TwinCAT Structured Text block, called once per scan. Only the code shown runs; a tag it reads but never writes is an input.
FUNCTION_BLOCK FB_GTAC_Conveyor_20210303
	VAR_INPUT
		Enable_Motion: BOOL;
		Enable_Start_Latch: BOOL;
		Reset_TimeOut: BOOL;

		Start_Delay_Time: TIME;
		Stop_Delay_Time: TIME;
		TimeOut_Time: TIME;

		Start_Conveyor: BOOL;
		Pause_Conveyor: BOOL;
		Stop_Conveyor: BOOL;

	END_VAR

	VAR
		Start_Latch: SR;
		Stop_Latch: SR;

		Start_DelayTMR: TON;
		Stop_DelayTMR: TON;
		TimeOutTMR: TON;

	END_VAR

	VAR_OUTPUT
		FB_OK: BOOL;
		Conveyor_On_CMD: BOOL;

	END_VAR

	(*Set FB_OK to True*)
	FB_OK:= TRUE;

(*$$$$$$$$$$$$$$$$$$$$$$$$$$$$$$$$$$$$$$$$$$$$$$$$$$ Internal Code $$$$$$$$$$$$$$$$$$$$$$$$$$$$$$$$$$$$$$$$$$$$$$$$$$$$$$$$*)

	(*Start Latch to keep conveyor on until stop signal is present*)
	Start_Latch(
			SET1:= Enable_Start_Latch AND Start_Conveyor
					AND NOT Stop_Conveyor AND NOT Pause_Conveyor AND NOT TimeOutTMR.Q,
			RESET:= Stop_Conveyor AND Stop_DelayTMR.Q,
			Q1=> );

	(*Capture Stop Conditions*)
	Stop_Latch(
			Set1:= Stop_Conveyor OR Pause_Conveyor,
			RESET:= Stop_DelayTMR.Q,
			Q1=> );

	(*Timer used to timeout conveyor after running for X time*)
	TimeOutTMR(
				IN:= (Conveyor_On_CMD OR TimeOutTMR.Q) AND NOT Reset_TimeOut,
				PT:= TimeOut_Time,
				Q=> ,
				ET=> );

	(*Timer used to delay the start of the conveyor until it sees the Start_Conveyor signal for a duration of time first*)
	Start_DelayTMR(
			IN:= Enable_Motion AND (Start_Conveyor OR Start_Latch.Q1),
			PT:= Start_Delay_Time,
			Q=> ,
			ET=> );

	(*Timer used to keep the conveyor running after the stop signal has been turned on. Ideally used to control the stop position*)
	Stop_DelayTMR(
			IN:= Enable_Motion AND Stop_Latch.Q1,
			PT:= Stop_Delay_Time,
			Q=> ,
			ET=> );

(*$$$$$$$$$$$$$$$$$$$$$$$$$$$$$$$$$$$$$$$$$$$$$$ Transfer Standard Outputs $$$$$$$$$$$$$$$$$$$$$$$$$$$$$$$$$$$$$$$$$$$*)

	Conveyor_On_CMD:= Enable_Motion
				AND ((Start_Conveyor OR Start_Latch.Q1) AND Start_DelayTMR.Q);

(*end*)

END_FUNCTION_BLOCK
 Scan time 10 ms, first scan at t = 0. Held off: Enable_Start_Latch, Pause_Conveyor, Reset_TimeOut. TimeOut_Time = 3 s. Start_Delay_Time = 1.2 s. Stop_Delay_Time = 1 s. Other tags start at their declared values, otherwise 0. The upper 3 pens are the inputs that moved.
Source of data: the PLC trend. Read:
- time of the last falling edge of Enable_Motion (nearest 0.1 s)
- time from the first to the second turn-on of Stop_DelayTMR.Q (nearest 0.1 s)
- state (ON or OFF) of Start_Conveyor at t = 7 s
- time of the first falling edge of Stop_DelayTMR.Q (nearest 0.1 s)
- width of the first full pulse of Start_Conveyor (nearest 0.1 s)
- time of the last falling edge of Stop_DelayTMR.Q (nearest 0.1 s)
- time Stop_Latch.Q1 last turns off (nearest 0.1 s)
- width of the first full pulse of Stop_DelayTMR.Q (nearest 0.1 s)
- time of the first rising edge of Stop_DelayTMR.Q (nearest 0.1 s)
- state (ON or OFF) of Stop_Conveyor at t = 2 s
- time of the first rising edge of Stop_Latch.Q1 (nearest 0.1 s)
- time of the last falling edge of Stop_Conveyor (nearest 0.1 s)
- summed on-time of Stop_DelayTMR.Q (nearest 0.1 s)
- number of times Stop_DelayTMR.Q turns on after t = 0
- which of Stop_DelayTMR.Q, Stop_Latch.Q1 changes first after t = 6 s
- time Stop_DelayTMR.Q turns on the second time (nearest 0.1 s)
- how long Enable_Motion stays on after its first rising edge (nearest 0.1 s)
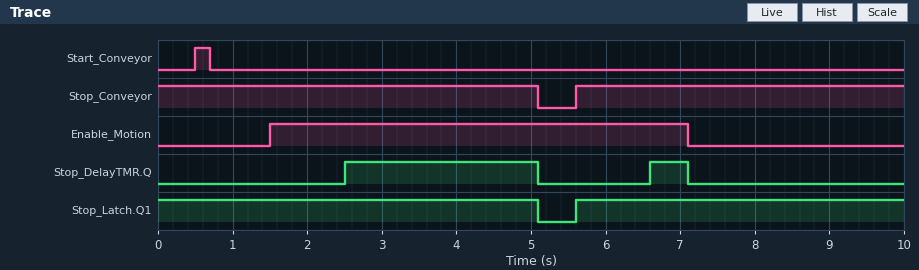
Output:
7.1 s
4.1 s
OFF
5.1 s
0.2 s
7.1 s
5.1 s
2.6 s
2.5 s
ON
5.6 s
5.1 s
3.1 s
2
Stop_DelayTMR.Q
6.6 s
5.6 s
